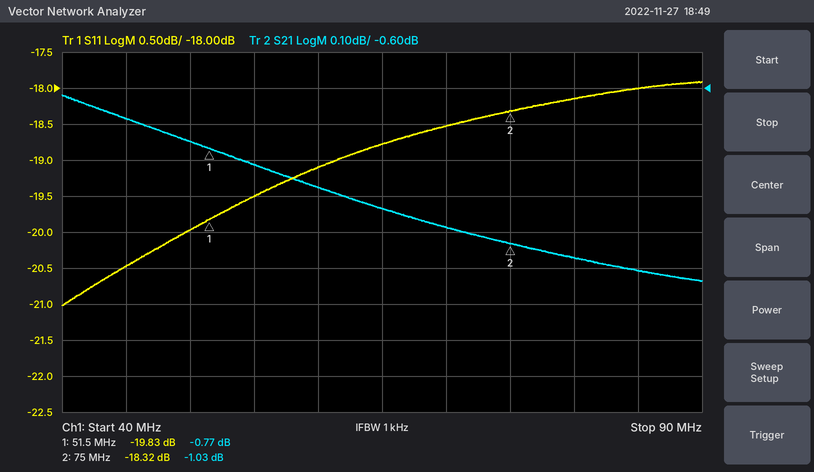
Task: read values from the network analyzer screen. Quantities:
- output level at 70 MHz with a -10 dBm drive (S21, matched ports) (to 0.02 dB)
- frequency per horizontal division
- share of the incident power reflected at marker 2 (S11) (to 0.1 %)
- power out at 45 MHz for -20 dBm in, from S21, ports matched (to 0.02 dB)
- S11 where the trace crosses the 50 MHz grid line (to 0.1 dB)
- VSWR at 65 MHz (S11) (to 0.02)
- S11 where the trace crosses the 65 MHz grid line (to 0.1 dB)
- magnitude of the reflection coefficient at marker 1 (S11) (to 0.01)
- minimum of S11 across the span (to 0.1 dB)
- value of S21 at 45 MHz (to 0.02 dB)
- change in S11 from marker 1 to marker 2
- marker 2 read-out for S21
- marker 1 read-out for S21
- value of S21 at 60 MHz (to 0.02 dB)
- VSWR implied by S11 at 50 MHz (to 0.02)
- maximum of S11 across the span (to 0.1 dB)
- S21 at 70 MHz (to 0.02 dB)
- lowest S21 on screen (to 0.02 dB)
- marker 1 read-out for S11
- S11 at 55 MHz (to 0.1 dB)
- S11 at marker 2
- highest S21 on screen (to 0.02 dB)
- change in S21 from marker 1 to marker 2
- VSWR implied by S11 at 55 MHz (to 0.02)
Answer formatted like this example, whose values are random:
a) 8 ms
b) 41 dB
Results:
a) -10.98 dBm
b) 5 MHz
c) 1.5 %
d) -20.68 dBm
e) -20.0 dB
f) 1.26
g) -18.8 dB
h) 0.10
i) -21.0 dB
j) -0.68 dB
k) 1.51 dB
l) -1.03 dB
m) -0.77 dB
n) -0.88 dB
o) 1.22
p) -17.9 dB
q) -0.98 dB
r) -1.14 dB
s) -19.83 dB
t) -19.5 dB
u) -18.32 dB
v) -0.62 dB
w) -0.26 dB
x) 1.24
